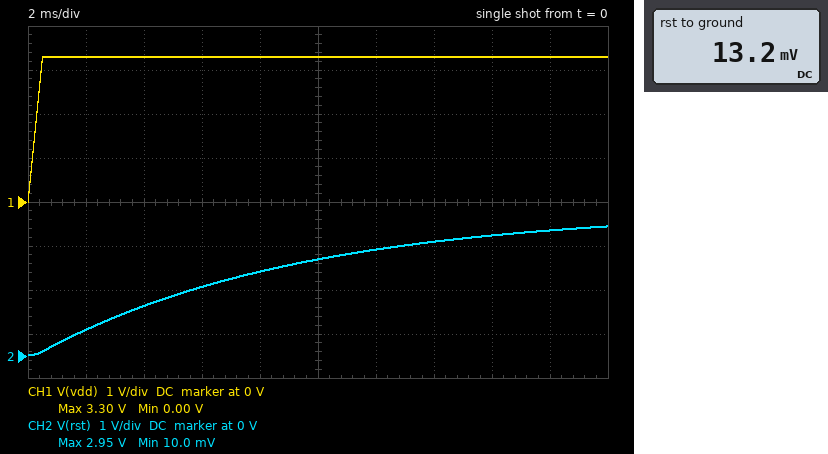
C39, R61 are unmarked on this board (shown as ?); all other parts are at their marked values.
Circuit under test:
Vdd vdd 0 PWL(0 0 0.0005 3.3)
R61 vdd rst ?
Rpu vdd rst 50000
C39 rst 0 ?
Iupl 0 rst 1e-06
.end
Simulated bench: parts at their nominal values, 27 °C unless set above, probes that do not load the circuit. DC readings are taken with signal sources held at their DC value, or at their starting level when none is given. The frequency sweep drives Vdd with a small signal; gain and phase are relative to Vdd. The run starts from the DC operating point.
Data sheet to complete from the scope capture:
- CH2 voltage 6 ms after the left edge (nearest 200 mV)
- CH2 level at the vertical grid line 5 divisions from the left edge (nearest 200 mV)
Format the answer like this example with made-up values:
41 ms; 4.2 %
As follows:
1.6 V; 2.2 V
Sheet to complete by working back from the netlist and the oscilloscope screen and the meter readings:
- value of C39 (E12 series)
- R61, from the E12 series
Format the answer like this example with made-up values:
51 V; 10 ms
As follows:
680 nF; 18 kΩ
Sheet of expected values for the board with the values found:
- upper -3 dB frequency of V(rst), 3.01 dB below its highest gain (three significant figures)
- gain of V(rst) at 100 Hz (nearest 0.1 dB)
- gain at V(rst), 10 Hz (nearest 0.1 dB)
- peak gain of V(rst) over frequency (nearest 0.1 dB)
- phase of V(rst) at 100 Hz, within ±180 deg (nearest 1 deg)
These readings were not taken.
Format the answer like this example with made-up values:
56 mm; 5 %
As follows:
17.7 Hz; -15.2 dB; -1.2 dB; 0 dB; -80 deg
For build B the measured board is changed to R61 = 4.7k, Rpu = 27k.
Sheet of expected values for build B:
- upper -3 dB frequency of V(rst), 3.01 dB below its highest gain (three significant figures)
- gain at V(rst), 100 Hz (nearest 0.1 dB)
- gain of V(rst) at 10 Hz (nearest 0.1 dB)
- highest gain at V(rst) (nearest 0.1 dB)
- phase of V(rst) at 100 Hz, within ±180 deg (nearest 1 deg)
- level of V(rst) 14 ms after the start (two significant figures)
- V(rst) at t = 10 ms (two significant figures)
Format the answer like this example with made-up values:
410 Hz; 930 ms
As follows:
58.5 Hz; -5.9 dB; -0.1 dB; 0 dB; -60 deg; 3.3 V; 3.2 V
